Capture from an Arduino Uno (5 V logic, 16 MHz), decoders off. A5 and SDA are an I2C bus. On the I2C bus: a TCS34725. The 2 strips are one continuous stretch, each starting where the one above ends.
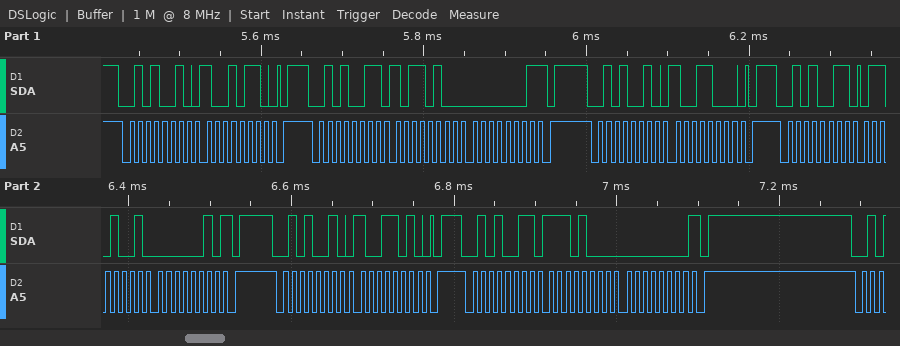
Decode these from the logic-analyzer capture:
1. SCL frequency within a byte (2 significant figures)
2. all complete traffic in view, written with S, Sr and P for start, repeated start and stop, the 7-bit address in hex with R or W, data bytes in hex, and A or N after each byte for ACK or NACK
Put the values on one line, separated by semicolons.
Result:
100 kHz; S 29W A 96 A P S 29R A B4 A 01 N P S 29W A 98 A P S 29R A 69 A 02 N P S 29W A 9A A P S 29R A E8 A 00 N P
